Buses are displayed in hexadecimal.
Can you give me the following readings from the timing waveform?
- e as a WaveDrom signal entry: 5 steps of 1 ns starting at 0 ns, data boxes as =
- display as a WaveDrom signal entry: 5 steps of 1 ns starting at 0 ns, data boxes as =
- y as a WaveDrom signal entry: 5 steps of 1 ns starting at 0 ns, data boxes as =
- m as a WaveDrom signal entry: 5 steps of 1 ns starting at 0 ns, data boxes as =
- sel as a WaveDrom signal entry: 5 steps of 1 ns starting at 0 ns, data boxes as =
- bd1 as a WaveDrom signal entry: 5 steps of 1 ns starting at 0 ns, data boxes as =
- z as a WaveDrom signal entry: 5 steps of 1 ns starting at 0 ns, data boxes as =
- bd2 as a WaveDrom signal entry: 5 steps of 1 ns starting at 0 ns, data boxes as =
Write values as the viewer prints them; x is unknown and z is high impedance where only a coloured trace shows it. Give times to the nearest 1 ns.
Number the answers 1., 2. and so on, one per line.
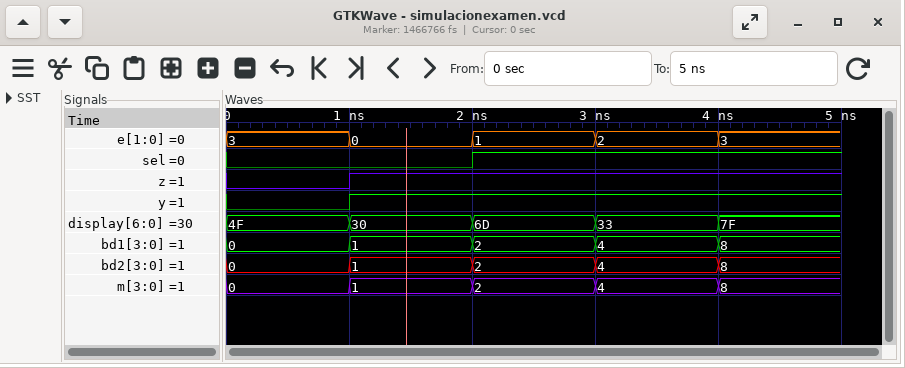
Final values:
1. {name: 'e', wave: '=====', data: '3 0 1 2 3'}
2. {name: 'display', wave: '=====', data: '4F 30 6D 33 7F'}
3. {name: 'y', wave: '01...'}
4. {name: 'm', wave: '=====', data: '0 1 2 4 8'}
5. {name: 'sel', wave: '0.1..'}
6. {name: 'bd1', wave: '=====', data: '0 1 2 4 8'}
7. {name: 'z', wave: '01...'}
8. {name: 'bd2', wave: '=====', data: '0 1 2 4 8'}
